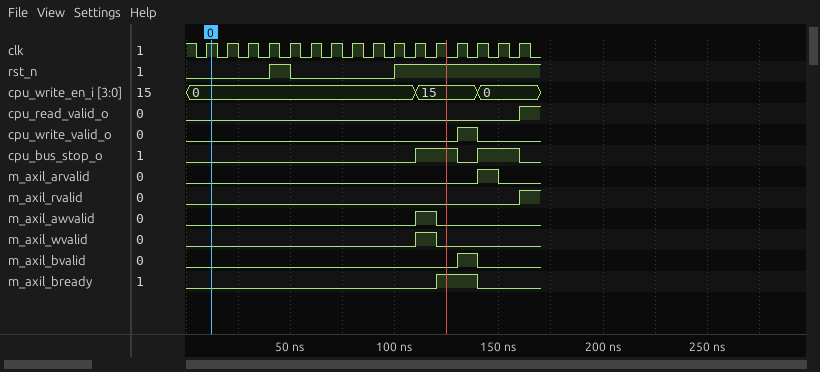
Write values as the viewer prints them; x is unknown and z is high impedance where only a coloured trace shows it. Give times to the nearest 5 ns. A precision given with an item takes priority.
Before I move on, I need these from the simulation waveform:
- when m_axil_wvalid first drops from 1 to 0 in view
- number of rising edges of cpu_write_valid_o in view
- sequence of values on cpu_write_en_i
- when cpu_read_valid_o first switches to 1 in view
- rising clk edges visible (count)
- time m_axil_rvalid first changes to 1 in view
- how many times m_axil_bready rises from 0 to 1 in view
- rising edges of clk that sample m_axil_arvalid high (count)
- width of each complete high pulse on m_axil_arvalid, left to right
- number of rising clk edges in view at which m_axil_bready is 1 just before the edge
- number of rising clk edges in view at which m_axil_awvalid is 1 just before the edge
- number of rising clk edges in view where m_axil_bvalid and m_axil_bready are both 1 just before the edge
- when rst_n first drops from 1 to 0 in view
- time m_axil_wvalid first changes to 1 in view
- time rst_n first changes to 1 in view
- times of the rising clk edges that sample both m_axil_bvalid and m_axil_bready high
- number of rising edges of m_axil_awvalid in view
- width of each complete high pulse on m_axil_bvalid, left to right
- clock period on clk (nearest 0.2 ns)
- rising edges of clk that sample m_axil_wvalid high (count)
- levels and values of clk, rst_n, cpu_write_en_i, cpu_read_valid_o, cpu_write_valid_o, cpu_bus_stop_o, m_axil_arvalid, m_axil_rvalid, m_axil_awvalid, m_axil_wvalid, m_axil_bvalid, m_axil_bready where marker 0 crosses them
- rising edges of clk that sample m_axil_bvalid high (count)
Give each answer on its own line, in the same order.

120 ns
1
0, 15, 0
160 ns
16
160 ns
1
1
10 ns
2
1
1
50 ns
110 ns
40 ns
140 ns
1
10 ns
10 ns
1
clk=1, rst_n=0, cpu_write_en_i=0, cpu_read_valid_o=0, cpu_write_valid_o=0, cpu_bus_stop_o=0, m_axil_arvalid=0, m_axil_rvalid=0, m_axil_awvalid=0, m_axil_wvalid=0, m_axil_bvalid=0, m_axil_bready=0
1
